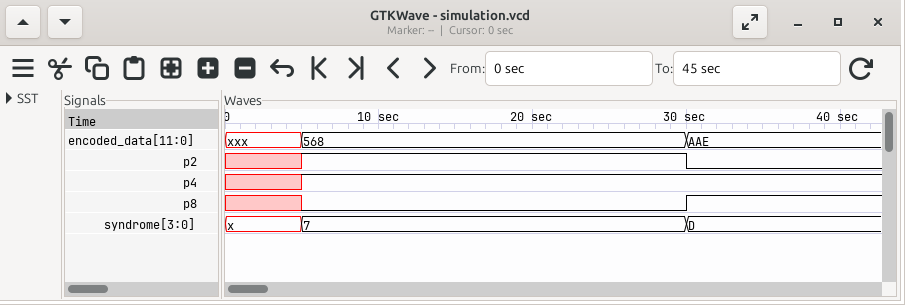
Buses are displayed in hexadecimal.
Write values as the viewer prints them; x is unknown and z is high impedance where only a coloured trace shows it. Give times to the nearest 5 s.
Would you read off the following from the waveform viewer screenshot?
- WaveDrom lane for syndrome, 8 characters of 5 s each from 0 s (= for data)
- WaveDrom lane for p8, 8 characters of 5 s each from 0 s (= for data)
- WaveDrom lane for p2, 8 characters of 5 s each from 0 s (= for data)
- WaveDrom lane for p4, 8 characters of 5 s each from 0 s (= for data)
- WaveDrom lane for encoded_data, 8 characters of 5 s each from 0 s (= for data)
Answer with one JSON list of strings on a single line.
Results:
["{name: 'syndrome', wave: 'x=....=.', data: '7 D'}", "{name: 'p8', wave: 'x0....1.'}", "{name: 'p2', wave: 'x1....0.'}", "{name: 'p4', wave: 'x1......'}", "{name: 'encoded_data', wave: 'x=....=.', data: '568 AAE'}"]
